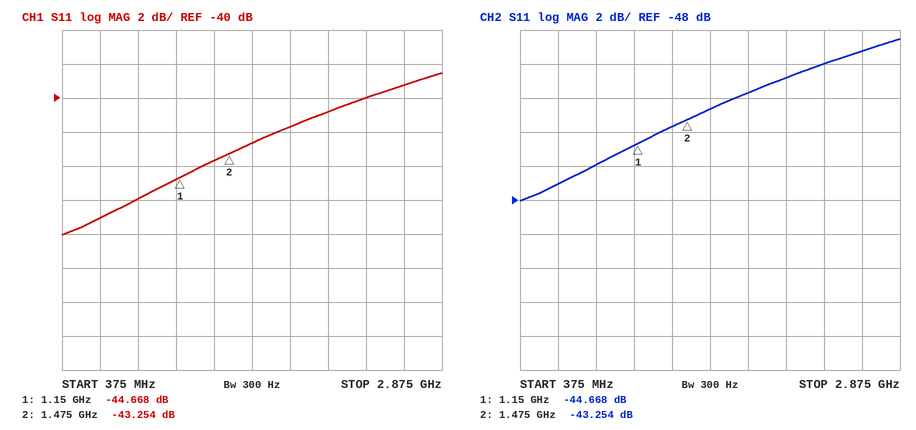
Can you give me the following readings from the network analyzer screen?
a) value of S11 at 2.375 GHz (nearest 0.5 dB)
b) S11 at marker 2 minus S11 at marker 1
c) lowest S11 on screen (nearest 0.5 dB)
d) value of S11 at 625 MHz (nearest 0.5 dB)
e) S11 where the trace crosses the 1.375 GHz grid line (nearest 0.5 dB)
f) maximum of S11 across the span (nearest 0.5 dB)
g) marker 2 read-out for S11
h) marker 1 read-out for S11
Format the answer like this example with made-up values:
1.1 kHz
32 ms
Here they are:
-40.0 dB
1.414 dB
-48.0 dB
-47.0 dB
-43.5 dB
-38.5 dB
-43.254 dB
-44.668 dB
